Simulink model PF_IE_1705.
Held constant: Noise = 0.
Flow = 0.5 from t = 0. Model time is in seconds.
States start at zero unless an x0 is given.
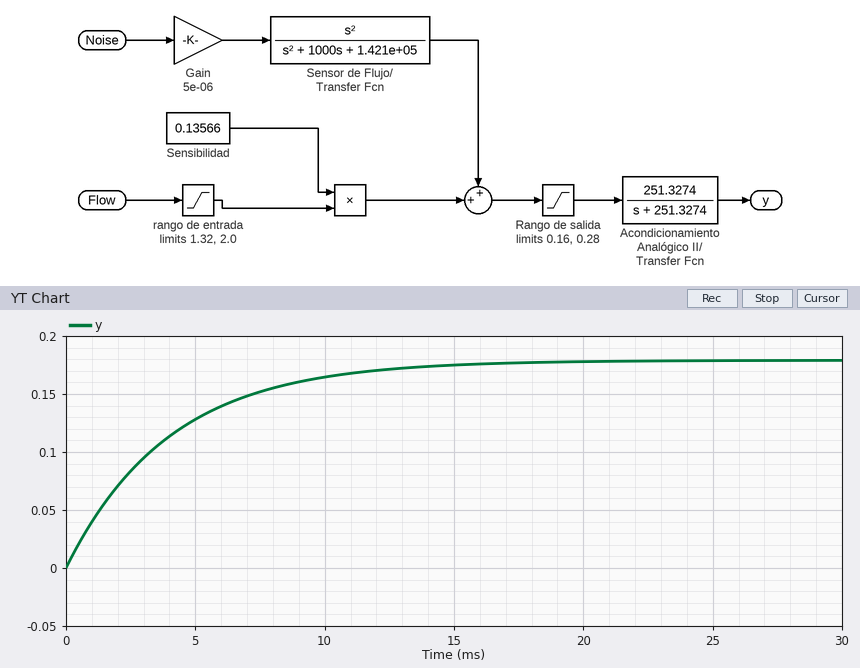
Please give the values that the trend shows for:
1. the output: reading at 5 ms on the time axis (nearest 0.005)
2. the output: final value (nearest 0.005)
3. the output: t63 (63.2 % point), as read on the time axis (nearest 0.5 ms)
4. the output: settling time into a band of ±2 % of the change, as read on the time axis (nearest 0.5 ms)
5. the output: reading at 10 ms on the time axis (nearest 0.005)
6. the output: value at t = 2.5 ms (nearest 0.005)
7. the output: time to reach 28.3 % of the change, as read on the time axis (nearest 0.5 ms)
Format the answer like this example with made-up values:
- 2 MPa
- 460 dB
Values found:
- 0.130
- 0.180
- 4.0 ms
- 15.5 ms
- 0.165
- 0.085
- 1.5 ms
